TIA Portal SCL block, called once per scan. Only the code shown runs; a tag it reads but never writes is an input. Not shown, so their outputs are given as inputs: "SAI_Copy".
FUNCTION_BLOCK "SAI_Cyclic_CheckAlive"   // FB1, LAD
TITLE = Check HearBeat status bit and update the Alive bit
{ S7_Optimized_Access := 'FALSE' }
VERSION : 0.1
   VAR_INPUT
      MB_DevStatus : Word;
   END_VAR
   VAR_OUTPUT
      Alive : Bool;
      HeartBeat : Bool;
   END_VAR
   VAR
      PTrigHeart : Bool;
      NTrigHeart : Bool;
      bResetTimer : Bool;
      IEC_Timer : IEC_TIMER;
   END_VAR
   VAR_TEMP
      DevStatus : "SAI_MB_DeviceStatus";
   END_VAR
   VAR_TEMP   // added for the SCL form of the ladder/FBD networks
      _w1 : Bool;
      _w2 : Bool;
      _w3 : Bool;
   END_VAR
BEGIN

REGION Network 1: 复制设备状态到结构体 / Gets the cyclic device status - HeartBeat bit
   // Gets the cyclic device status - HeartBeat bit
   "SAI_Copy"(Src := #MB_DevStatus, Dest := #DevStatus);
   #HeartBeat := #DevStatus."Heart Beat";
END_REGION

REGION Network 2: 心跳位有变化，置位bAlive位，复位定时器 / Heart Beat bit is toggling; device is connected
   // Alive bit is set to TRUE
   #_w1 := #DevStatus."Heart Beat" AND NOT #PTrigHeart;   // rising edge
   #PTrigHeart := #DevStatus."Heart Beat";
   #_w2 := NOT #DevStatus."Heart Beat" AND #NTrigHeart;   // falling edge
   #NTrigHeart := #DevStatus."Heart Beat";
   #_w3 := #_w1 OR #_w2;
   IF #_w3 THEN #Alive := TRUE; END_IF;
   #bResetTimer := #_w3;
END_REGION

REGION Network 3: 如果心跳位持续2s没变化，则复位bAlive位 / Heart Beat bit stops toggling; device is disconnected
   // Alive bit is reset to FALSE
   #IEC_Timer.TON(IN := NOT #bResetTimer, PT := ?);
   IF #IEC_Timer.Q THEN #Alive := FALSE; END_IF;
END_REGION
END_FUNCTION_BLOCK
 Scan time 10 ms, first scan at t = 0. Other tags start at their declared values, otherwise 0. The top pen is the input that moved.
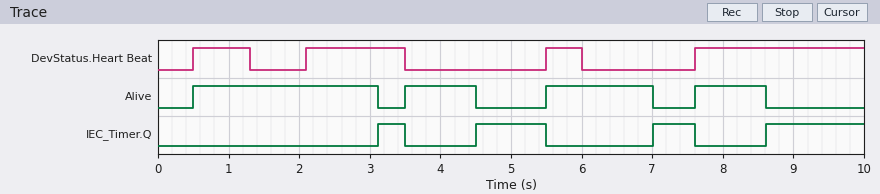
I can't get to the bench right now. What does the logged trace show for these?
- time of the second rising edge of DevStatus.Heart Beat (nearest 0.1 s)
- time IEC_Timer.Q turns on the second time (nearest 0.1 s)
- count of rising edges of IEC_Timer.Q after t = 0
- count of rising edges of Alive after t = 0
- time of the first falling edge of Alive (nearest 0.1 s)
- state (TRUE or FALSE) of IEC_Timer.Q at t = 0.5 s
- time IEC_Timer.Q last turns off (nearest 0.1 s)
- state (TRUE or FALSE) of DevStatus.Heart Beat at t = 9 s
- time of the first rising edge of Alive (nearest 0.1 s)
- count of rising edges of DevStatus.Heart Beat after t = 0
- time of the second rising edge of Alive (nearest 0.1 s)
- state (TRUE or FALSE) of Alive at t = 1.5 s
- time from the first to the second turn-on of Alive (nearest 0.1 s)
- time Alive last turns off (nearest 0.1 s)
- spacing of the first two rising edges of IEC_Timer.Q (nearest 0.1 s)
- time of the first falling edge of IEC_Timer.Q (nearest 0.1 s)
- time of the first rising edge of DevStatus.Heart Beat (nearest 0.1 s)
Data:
2.1 s
4.5 s
4
4
3.1 s
FALSE
7.6 s
TRUE
0.5 s
4
3.5 s
TRUE
3.0 s
8.6 s
1.4 s
3.5 s
0.5 s
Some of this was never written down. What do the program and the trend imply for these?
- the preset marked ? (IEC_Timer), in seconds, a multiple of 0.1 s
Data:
1.0 s
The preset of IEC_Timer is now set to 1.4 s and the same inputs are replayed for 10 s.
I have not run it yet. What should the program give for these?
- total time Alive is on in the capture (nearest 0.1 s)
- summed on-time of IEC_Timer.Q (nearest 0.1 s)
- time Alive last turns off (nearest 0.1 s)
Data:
7.7 s
1.8 s
9.0 s
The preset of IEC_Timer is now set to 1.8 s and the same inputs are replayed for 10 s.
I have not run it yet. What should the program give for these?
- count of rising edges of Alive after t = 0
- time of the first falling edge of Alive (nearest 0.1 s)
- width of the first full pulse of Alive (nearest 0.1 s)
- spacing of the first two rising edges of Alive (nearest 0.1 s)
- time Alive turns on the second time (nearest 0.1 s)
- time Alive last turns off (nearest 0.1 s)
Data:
2
5.3 s
4.8 s
5.0 s
5.5 s
9.4 s
